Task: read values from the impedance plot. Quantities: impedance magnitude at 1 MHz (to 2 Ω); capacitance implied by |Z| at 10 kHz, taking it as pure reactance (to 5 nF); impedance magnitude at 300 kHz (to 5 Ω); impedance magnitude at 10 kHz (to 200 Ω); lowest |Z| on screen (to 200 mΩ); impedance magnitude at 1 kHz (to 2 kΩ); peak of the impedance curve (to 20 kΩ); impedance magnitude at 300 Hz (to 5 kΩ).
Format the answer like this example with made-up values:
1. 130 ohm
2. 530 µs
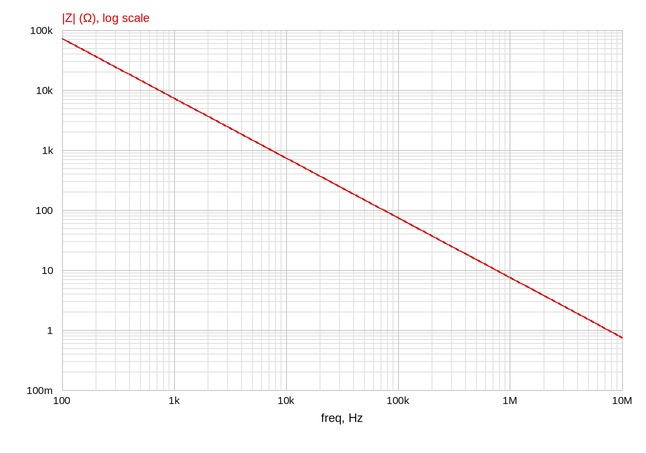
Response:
1. 8 Ω
2. 20 nF
3. 25 Ω
4. 800 Ω
5. 800 mΩ
6. 8 kΩ
7. 80 kΩ
8. 25 kΩ
